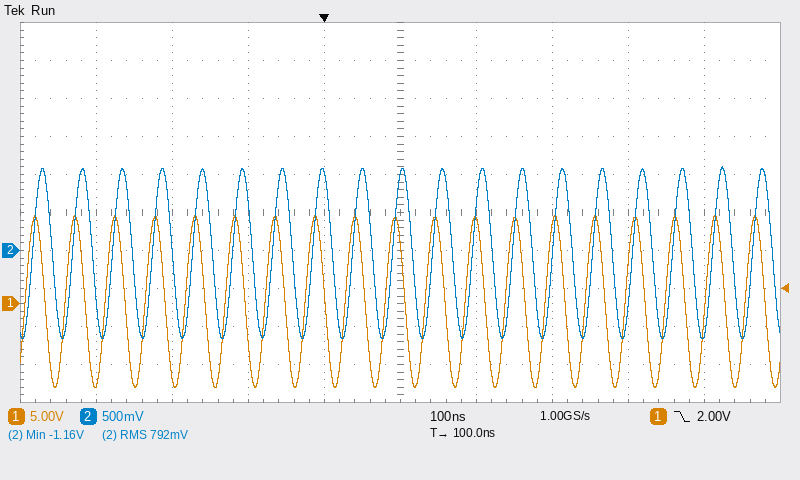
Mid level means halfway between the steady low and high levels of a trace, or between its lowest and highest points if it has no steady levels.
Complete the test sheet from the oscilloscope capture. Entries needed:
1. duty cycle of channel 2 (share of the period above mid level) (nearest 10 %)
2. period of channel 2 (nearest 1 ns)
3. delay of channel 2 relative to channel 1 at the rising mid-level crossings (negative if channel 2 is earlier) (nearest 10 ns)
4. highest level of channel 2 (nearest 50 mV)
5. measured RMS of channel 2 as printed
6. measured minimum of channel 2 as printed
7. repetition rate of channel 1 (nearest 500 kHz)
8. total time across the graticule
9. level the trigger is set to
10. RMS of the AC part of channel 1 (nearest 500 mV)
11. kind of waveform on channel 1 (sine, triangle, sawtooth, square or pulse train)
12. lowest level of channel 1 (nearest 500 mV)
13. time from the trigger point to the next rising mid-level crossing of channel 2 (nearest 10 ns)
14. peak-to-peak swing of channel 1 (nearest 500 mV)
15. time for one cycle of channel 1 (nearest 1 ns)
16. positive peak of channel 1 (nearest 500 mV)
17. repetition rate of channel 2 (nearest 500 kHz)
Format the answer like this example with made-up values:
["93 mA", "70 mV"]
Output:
["50 %", "53 ns", "+10 ns", "1.10 V", "792 mV", "-1.16 V", "19.0 MHz", "1 µs", "2.00 V", "8.0 V", "sine", "-11.0 V", "40 ns", "22.5 V", "53 ns", "11.5 V", "19.0 MHz"]
